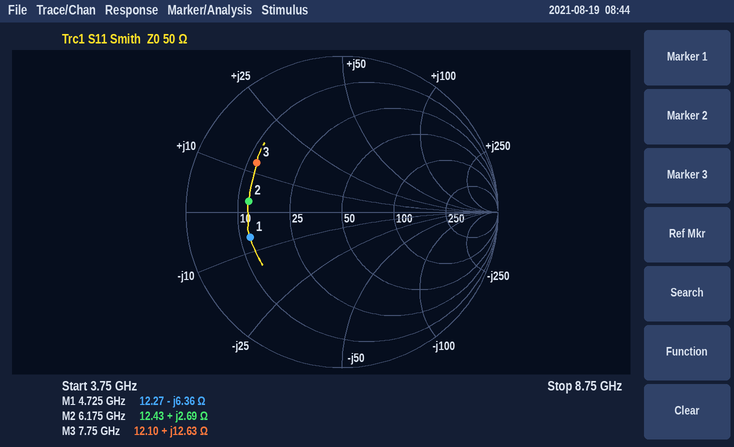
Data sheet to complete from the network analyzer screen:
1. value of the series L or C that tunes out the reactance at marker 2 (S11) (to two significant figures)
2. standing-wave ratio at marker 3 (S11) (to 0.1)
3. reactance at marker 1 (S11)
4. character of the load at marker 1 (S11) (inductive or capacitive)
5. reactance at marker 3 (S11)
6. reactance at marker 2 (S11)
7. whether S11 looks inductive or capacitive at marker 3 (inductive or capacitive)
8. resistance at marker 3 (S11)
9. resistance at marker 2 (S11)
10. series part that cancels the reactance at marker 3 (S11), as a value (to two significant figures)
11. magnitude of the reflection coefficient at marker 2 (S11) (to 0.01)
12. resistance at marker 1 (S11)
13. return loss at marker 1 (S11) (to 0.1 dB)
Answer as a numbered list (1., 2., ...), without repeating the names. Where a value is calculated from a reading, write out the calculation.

1. C = 1/(2π × 6.175 GHz × 2.69 Ω) ≈ 9.6 pF
2. 4.4
3. -6.36 Ω
4. capacitive
5. +12.63 Ω
6. +2.69 Ω
7. inductive
8. 12.10 Ω
9. 12.43 Ω
10. C = 1/(2π × 7.75 GHz × 12.63 Ω) ≈ 1.6 pF
11. 0.60
12. 12.27 Ω
13. 4.3 dB
